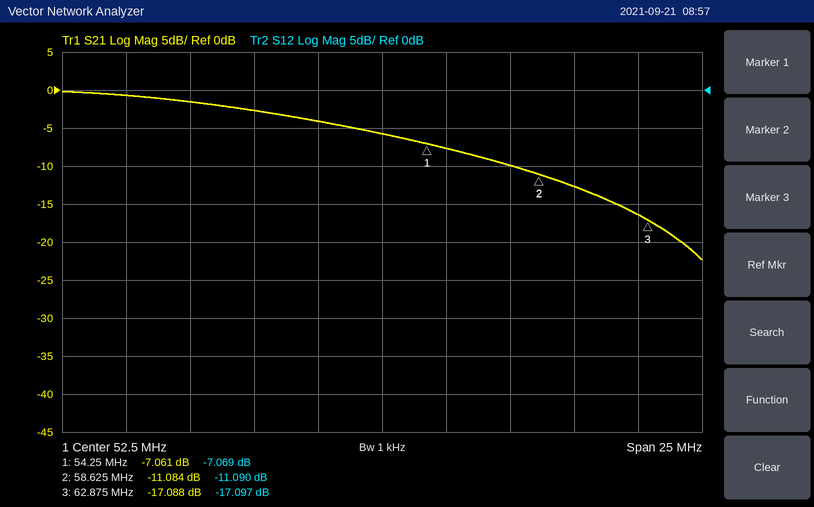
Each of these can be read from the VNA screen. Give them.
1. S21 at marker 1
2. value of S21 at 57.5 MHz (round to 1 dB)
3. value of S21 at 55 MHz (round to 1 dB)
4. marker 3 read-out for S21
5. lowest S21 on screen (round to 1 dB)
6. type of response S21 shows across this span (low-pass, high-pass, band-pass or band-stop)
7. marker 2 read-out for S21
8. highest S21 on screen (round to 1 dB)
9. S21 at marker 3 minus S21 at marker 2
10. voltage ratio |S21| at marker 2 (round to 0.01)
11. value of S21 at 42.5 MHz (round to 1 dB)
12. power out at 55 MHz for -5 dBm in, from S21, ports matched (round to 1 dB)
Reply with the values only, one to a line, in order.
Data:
-7.061 dB
-10 dB
-8 dB
-17.088 dB
-22 dB
low-pass
-11.084 dB
0 dB
-6.004 dB
0.28
-1 dB
-13 dBm
